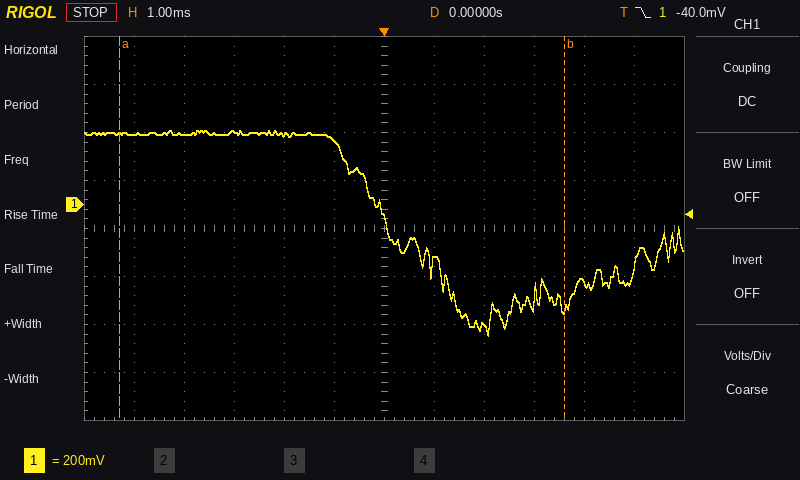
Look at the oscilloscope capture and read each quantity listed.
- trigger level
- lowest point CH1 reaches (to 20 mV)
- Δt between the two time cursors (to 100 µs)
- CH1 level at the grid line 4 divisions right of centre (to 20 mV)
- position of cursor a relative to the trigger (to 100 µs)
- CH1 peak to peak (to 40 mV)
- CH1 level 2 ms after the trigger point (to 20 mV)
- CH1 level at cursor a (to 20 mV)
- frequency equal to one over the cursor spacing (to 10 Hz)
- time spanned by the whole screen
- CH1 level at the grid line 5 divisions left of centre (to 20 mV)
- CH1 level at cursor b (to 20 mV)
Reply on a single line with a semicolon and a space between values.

-40.0 mV; -540 mV; 8.9 ms; -320 mV; -5.3 ms; 840 mV; -500 mV; 300 mV; 110 Hz; 12 ms; 300 mV; -440 mV
